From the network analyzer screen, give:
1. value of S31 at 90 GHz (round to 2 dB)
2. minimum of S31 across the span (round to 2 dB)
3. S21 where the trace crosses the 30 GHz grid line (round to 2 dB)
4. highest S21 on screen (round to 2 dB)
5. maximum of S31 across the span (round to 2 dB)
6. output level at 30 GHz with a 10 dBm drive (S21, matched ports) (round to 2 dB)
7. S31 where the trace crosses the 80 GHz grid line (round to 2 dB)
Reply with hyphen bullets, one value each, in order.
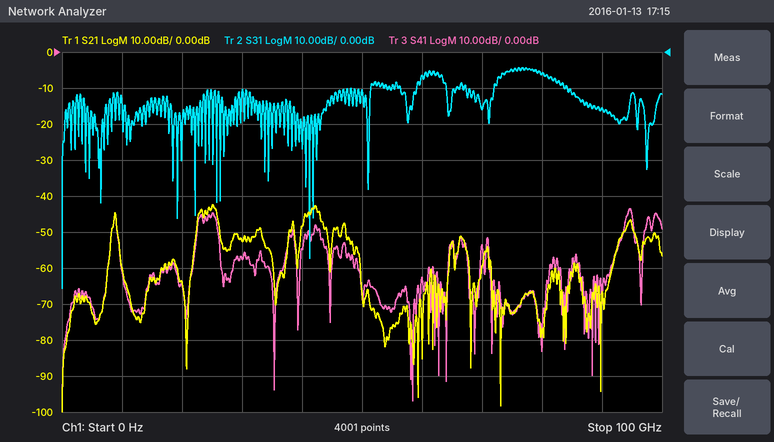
- -16 dB
- -66 dB
- -52 dB
- -42 dB
- -4 dB
- -42 dBm
- -6 dB
